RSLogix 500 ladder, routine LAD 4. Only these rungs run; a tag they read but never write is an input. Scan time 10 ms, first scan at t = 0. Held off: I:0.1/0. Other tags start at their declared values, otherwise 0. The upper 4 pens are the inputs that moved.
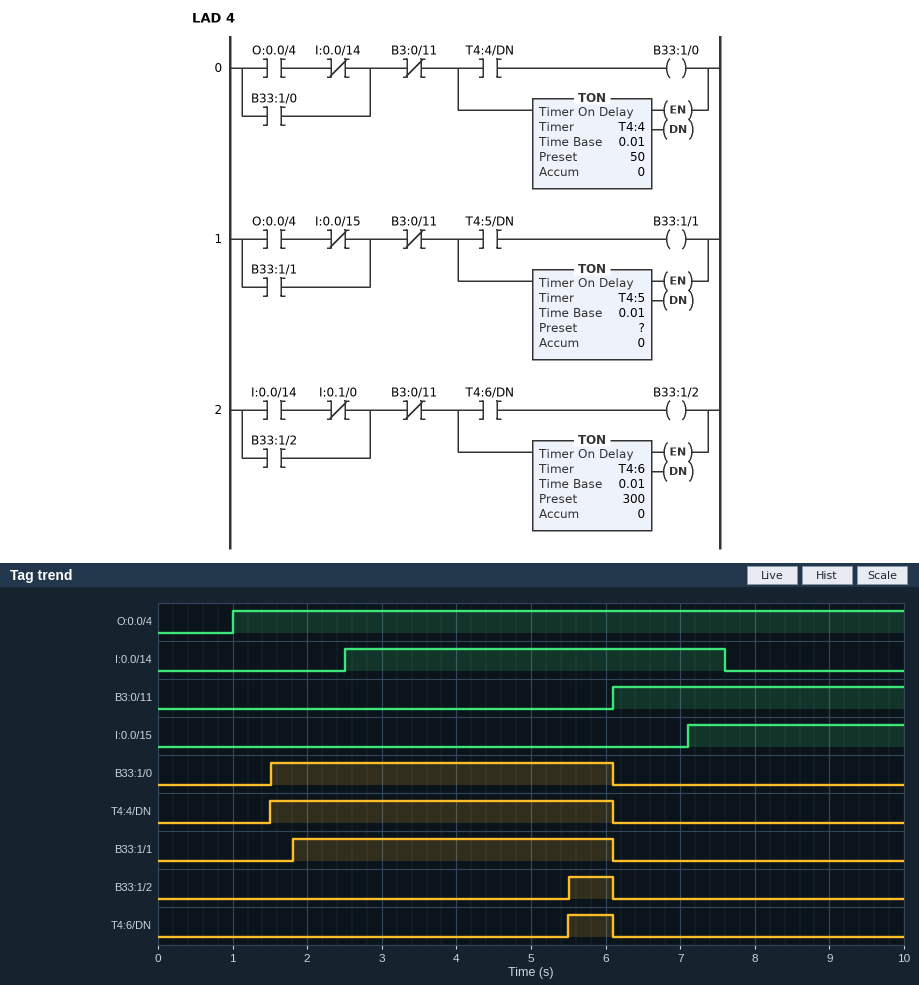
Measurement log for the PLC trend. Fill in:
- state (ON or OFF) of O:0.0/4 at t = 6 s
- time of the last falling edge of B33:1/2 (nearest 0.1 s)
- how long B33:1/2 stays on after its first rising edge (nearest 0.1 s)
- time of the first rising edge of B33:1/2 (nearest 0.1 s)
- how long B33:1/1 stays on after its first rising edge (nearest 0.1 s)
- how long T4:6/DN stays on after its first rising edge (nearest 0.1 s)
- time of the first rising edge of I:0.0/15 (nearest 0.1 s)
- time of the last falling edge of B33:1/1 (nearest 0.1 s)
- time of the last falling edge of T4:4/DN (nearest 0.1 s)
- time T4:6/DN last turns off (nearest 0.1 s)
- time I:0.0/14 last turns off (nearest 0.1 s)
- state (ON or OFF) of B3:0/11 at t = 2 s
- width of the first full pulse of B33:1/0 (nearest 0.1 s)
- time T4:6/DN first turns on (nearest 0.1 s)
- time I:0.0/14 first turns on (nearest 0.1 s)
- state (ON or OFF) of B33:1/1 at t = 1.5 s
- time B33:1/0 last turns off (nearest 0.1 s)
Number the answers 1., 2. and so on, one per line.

1. ON
2. 6.1 s
3. 0.6 s
4. 5.5 s
5. 4.3 s
6. 0.6 s
7. 7.1 s
8. 6.1 s
9. 6.1 s
10. 6.1 s
11. 7.6 s
12. OFF
13. 4.6 s
14. 5.5 s
15. 2.5 s
16. OFF
17. 6.1 s
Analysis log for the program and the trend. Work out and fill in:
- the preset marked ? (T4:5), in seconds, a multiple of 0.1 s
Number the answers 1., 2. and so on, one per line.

1. 0.8 s
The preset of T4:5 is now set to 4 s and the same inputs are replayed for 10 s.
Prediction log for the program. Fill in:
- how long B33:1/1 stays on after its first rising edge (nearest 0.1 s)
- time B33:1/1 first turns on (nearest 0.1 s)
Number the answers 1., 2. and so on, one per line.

1. 1.1 s
2. 5.0 s
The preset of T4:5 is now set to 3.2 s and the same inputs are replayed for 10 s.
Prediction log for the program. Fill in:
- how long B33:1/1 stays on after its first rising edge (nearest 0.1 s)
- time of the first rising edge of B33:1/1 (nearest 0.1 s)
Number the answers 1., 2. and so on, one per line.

1. 1.9 s
2. 4.2 s
